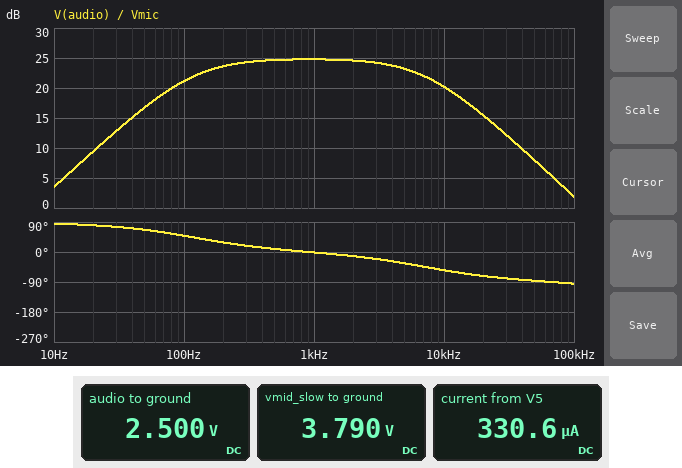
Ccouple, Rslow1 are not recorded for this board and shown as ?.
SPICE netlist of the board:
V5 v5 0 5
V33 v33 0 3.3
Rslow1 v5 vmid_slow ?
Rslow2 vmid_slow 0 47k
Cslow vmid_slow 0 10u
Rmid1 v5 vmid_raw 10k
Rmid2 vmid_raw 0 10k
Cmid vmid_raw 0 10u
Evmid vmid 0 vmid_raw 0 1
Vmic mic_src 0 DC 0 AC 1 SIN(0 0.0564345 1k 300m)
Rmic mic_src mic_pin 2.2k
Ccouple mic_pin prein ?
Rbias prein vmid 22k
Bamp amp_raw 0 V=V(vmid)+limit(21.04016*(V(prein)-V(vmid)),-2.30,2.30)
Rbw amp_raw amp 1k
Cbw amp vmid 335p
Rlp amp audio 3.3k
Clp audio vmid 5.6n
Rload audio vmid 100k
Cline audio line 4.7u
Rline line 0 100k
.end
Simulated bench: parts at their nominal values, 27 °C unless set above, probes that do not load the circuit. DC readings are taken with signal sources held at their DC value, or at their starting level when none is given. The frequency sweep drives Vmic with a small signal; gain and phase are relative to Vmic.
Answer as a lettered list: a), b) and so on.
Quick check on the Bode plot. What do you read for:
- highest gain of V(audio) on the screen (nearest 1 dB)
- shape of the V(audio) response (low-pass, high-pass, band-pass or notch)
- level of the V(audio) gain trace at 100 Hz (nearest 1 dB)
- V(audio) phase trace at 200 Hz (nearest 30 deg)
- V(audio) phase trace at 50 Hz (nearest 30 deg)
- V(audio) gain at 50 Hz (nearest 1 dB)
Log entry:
a) 25 dB
b) band-pass
c) 21 dB
d) 30 deg
e) 60 deg
f) 17 dB
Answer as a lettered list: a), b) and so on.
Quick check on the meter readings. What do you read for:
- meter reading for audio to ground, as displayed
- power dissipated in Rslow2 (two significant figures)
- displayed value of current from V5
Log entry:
a) 2.500 V
b) 310 µW
c) 330.6 µA
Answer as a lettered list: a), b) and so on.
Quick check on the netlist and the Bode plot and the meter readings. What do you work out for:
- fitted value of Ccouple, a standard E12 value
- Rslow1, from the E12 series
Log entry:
a) 56 nF
b) 15 kΩ
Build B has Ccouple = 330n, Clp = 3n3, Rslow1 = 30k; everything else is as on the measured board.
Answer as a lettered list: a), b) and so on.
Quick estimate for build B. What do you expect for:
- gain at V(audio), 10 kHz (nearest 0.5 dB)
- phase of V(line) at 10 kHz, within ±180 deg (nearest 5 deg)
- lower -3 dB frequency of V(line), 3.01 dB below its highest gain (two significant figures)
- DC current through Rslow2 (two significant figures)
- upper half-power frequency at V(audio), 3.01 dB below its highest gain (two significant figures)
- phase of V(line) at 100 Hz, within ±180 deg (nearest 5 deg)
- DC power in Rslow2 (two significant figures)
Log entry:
a) 22.5 dB
b) -40 deg
c) 20 Hz
d) 65 µA
e) 12 kHz
f) 10 deg
g) 200 µW
